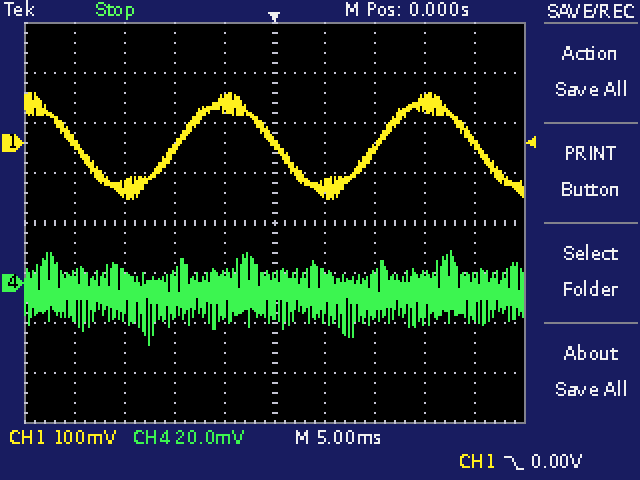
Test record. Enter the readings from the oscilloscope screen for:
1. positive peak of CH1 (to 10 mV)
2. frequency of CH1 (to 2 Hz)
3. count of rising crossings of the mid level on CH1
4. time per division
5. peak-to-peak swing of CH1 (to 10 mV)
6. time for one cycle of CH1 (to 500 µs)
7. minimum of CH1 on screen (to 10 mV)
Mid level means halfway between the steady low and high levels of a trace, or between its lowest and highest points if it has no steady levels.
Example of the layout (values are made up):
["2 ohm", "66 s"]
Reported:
["100 mV", "50 Hz", "2", "5 ms", "210 mV", "20.0 ms", "-110 mV"]
